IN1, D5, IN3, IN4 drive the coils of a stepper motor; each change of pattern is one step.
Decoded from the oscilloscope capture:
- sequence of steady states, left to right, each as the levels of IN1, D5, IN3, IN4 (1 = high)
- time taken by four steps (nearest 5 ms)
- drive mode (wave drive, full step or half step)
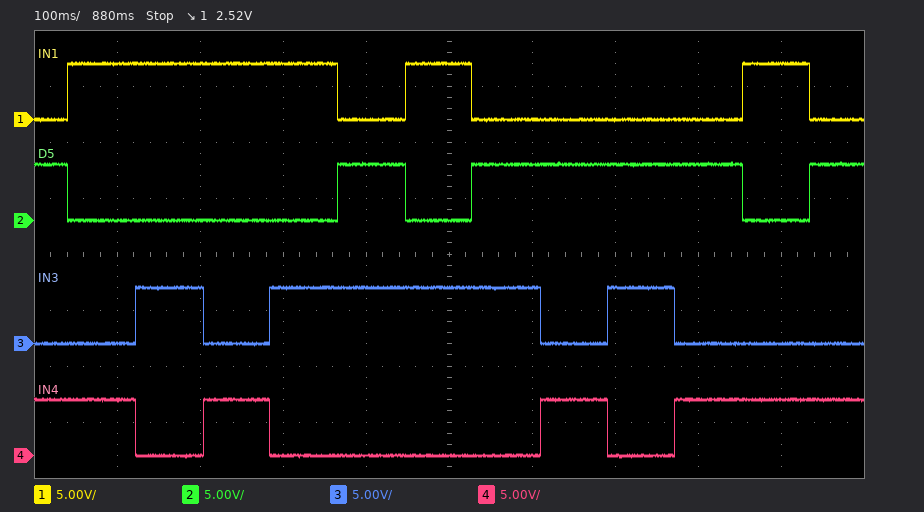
0101 1001 1010 1001 1010 0110 1010 0110 0101 0110 0101 1001 0101
325 ms
full step
